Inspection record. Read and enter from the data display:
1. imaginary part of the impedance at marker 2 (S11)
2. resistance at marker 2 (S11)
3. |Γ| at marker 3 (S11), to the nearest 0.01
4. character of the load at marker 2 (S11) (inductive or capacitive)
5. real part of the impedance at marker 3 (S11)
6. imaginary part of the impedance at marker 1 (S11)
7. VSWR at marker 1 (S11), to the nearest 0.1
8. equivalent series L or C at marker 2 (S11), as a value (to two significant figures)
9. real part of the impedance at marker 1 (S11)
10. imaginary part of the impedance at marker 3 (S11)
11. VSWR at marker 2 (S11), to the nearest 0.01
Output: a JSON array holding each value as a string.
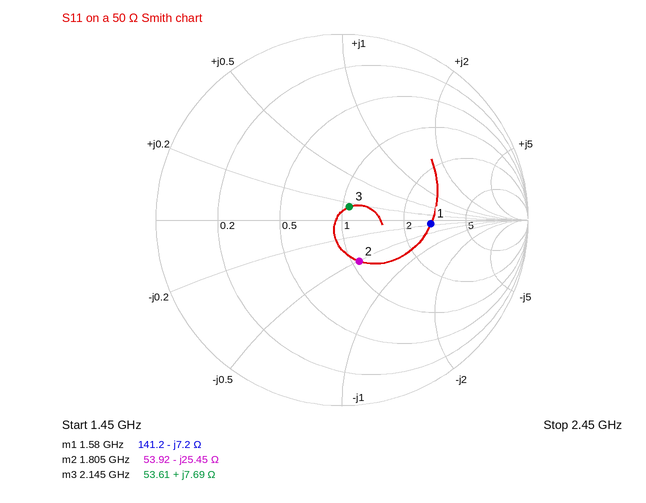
["-25.45 Ω", "53.92 Ω", "0.08", "capacitive", "53.61 Ω", "-7.2 Ω", "2.8", "3.5 pF", "141.2 Ω", "+7.69 Ω", "1.63"]
